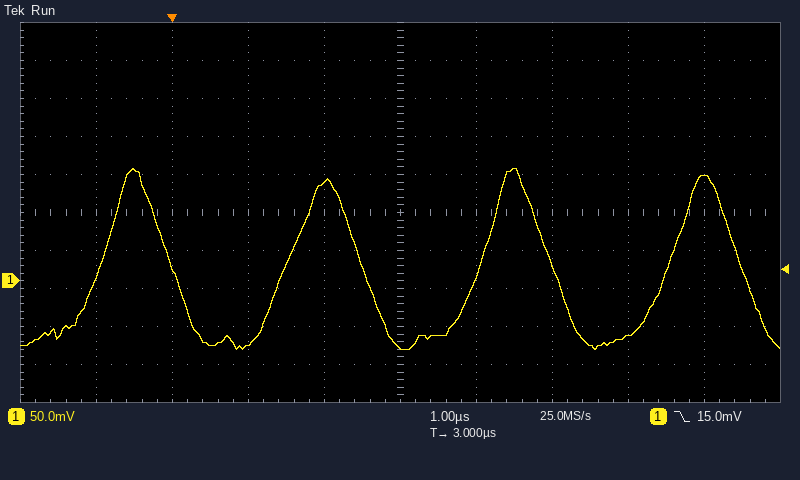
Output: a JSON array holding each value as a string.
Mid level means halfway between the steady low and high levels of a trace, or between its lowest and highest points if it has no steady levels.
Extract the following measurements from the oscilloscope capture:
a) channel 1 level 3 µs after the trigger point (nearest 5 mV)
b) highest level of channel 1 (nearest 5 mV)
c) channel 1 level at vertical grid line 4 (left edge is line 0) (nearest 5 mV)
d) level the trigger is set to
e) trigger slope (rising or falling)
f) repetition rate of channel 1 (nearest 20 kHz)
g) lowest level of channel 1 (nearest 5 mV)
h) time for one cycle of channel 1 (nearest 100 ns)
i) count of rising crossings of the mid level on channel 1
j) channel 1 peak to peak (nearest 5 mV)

["-85 mV", "150 mV", "130 mV", "15.0 mV", "falling", "400 kHz", "-90 mV", "2.5 µs", "4", "240 mV"]
